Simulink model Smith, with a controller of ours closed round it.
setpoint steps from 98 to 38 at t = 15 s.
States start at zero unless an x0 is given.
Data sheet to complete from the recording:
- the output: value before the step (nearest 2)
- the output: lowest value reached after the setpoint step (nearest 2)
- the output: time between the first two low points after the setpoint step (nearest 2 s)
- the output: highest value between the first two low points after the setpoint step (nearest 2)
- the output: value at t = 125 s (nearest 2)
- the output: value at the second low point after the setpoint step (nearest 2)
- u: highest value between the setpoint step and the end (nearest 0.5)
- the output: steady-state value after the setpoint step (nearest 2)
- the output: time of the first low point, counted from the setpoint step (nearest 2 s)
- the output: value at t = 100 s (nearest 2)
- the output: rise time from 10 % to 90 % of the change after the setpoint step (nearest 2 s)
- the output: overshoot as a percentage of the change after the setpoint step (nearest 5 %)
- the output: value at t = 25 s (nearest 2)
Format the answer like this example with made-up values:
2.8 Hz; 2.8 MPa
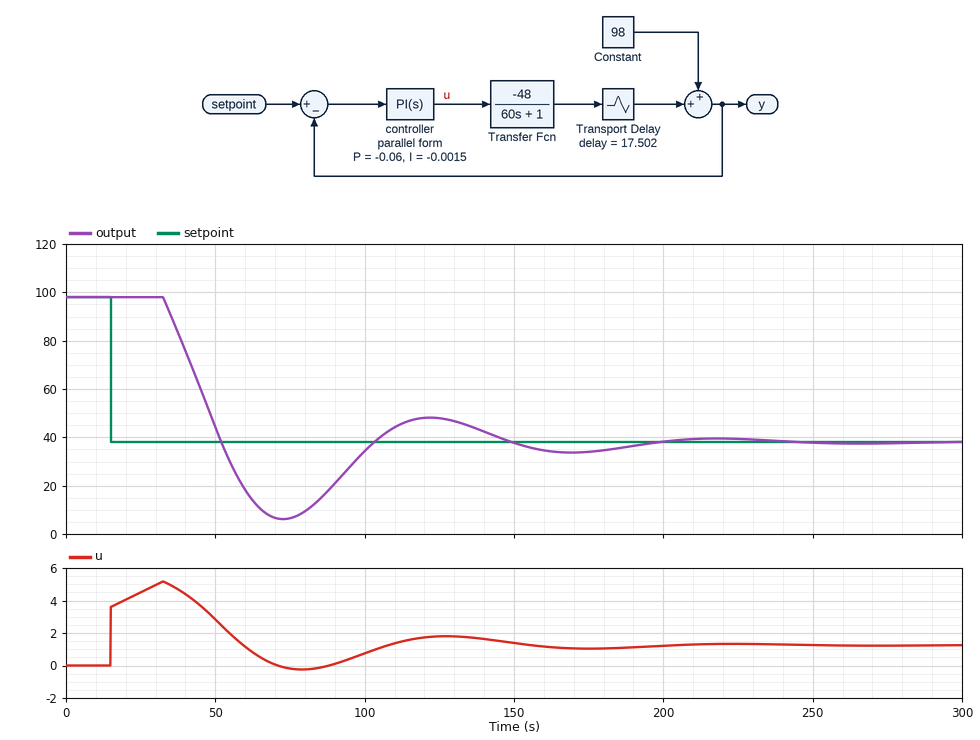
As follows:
98; 6; 96 s; 48; 48; 34; 5.0; 38; 58 s; 34; 16 s; 55 %; 98
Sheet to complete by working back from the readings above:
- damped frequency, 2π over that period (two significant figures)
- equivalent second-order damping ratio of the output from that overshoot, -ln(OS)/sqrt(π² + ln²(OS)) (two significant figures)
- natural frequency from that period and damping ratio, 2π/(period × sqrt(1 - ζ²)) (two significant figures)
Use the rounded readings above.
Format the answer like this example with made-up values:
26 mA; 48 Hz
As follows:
0.065 rad/s; 0.19; 0.067 rad/s
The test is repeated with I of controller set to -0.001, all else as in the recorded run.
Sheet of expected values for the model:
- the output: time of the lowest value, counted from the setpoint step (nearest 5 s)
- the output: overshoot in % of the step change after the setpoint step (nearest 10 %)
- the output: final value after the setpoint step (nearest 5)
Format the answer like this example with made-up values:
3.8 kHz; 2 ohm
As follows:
55 s; 30 %; 40
